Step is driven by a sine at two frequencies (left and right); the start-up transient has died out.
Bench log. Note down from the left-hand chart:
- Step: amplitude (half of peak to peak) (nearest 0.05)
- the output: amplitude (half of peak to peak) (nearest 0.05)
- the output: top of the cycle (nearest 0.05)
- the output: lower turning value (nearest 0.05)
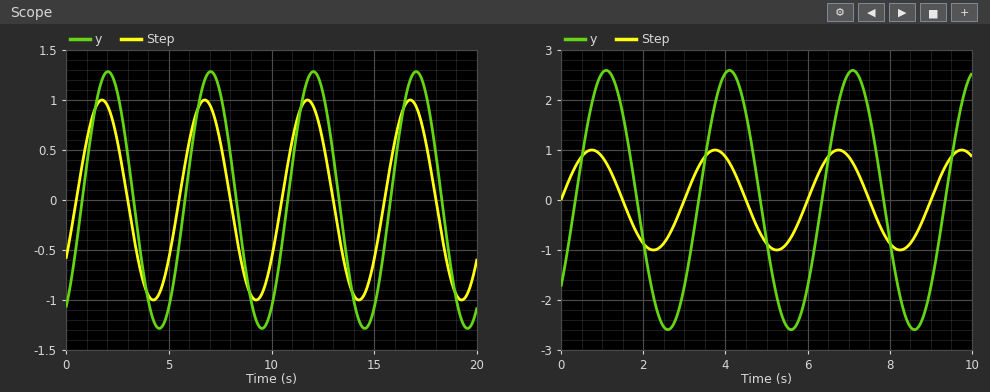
1.00
1.30
1.30
-1.30
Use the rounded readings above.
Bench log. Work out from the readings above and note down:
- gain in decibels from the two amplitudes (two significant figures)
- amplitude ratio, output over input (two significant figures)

2.3 dB
1.3
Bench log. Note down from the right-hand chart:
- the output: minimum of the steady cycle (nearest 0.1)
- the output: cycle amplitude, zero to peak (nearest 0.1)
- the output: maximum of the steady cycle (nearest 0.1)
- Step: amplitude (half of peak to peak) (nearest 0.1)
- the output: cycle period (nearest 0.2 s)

-2.6
2.6
2.6
1.0
3.0 s
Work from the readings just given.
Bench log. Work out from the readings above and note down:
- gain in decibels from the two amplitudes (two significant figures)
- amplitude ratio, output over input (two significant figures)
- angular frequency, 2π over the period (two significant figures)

8.3 dB
2.6
2.1 rad/s
